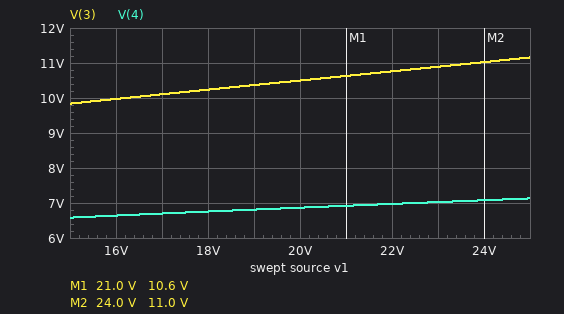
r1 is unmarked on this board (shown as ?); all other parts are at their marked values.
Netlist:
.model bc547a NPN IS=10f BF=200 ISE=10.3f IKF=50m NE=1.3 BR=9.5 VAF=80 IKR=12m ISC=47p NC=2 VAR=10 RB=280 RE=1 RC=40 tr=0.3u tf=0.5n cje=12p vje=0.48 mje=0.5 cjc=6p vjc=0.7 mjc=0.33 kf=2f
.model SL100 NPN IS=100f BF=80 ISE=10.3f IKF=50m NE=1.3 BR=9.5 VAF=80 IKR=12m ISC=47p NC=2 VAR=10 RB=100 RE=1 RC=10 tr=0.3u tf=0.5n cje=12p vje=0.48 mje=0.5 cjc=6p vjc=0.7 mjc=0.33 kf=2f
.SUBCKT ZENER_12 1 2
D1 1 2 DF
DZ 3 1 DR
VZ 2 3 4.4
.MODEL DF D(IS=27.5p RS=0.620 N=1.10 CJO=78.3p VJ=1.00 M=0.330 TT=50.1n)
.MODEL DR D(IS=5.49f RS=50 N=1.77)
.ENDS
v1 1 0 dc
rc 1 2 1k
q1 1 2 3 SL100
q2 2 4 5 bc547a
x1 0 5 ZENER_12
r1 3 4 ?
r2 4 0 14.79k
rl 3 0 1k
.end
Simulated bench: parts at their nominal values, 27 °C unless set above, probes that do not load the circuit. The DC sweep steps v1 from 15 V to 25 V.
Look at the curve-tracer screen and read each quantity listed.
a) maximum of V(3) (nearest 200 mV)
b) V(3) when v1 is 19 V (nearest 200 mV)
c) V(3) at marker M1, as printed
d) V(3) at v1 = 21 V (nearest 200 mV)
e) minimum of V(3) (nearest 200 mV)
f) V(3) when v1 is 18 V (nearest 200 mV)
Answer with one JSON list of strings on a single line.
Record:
["11.2 V", "10.4 V", "10.6 V", "10.6 V", "9.8 V", "10.2 V"]
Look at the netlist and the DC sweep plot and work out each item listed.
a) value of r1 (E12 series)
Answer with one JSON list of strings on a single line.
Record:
["6.8 kΩ"]
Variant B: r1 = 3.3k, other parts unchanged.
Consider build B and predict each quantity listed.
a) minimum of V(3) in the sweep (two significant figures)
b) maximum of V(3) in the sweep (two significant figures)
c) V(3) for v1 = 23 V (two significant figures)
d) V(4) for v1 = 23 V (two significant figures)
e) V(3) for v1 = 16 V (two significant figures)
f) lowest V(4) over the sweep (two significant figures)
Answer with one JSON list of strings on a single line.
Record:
["8.3 V", "9.3 V", "9.1 V", "7.1 V", "8.4 V", "6.7 V"]
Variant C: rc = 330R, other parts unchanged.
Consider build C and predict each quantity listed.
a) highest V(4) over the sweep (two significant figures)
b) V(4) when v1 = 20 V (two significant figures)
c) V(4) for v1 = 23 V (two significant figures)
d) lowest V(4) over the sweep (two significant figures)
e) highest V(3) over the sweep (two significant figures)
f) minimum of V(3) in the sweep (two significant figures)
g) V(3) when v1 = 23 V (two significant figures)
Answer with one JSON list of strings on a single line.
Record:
["8.2 V", "7.6 V", "7.9 V", "7.0 V", "14 V", "11 V", "13 V"]
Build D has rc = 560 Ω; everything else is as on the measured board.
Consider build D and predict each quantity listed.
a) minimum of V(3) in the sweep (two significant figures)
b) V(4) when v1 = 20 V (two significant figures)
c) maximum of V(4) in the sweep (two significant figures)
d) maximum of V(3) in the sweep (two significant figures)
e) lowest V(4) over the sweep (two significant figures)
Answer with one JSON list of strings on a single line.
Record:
["10 V", "7.2 V", "7.6 V", "12 V", "6.8 V"]
